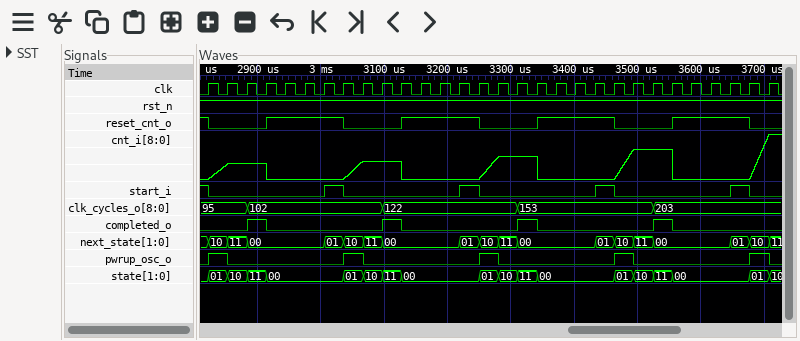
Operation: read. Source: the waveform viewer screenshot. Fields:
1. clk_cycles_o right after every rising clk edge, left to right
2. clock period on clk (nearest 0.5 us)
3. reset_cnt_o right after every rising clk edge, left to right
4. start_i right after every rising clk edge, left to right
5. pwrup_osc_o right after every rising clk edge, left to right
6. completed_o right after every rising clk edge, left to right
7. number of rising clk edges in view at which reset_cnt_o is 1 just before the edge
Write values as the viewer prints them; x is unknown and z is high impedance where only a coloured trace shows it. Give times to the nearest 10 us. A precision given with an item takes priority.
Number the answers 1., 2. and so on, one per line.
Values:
1. 95, 95, 102, 102, 102, 102, 102, 102, 102, 122, 122, 122, 122, 122, 122, 122, 153, 153, 153, 153, 153, 153, 153, 203, 203, 203, 203, 203, 203, 203
2. 30.5 us
3. 0 0 0 1 1 1 1 0 0 0 1 1 1 1 0 0 0 1 1 1 1 0 0 0 1 1 1 1 0 0
4. 0 0 0 0 0 0 1 0 0 0 0 0 0 1 0 0 0 0 0 0 1 0 0 0 0 0 0 1 0 0
5. 1 0 0 0 0 0 0 1 0 0 0 0 0 0 1 0 0 0 0 0 0 1 0 0 0 0 0 0 1 0
6. 0 0 1 0 0 0 0 0 0 1 0 0 0 0 0 0 1 0 0 0 0 0 0 1 0 0 0 0 0 0
7. 17
